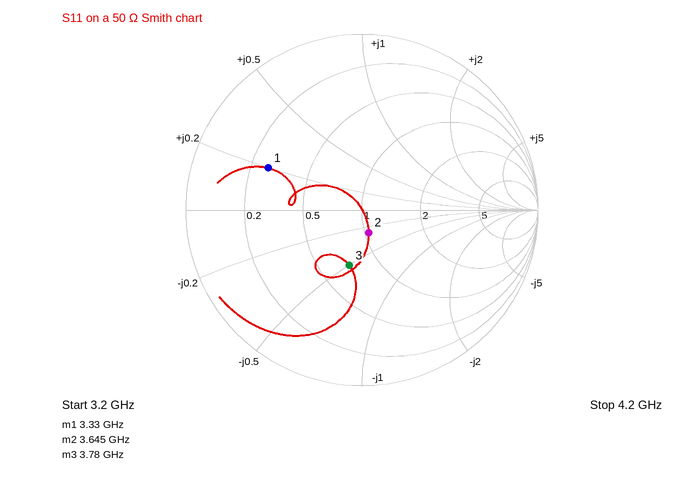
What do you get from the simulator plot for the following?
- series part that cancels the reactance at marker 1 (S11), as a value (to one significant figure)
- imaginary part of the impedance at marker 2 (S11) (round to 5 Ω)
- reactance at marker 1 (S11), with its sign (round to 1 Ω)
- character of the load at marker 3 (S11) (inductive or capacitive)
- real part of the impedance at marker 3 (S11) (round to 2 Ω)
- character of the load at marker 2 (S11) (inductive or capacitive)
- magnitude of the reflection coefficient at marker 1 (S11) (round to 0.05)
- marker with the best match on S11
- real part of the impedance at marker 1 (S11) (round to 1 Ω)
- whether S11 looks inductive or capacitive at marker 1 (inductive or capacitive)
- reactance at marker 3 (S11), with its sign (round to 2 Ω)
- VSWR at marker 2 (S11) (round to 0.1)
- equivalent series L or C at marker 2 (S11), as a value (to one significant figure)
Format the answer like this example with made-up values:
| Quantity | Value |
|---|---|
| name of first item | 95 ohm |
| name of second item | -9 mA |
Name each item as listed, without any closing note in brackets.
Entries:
| Quantity | Value |
|---|---|
| series part that cancels the reactance at marker 1 (S11), as a value | 5 pF |
| imaginary part of the impedance at marker 2 (S11) | -15 Ω |
| reactance at marker 1 (S11), with its sign | +10 Ω |
| character of the load at marker 3 (S11) | capacitive |
| real part of the impedance at marker 3 (S11) | 36 Ω |
| character of the load at marker 2 (S11) | capacitive |
| magnitude of the reflection coefficient at marker 1 (S11) | 0.60 |
| marker with the best match on S11 | marker 2 |
| real part of the impedance at marker 1 (S11) | 14 Ω |
| whether S11 looks inductive or capacitive at marker 1 | inductive |
| reactance at marker 3 (S11), with its sign | -26 Ω |
| VSWR at marker 2 (S11) | 1.3 |
| equivalent series L or C at marker 2 (S11), as a value | 3 pF |
